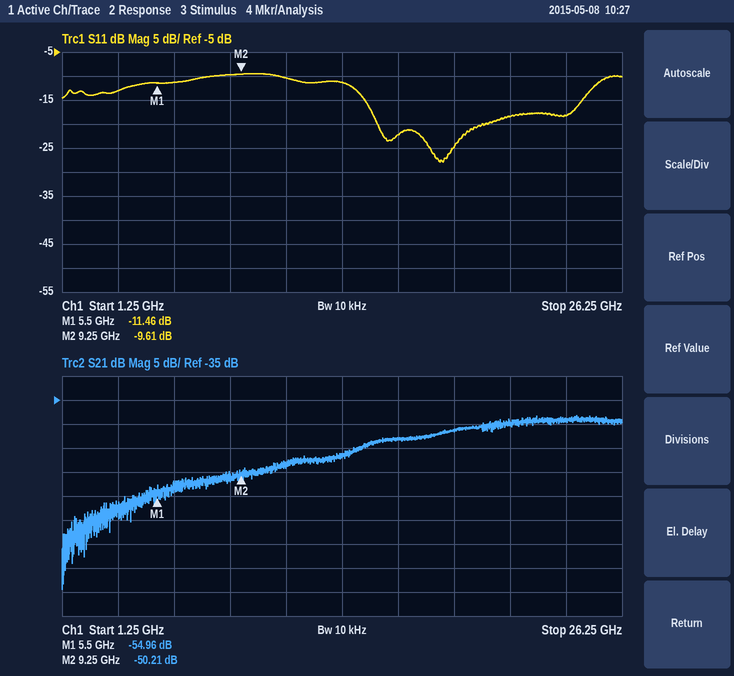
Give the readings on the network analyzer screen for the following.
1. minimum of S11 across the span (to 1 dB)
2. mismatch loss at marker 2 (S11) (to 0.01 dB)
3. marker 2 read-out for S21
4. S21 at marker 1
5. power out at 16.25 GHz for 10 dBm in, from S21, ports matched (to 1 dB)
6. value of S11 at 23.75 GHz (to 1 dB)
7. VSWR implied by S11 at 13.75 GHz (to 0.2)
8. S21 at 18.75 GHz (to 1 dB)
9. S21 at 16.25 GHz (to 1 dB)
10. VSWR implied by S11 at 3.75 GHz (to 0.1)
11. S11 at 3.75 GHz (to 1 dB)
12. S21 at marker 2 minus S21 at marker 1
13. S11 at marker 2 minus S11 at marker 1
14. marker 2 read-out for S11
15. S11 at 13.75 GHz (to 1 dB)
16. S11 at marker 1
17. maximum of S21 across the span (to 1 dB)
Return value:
-28 dB
0.50 dB
-50.21 dB
-54.96 dB
-33 dBm
-18 dB
1.8
-41 dB
-43 dB
1.6
-13 dB
4.75 dB
1.85 dB
-9.61 dB
-11 dB
-11.46 dB
-38 dB
